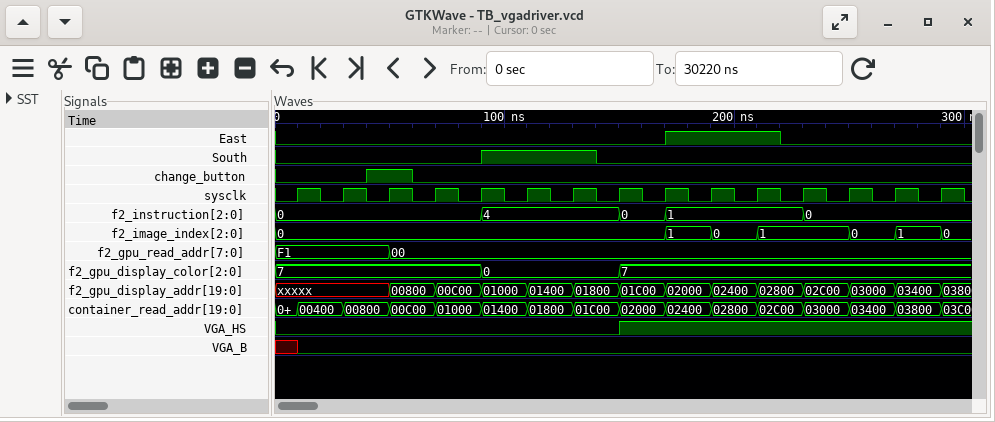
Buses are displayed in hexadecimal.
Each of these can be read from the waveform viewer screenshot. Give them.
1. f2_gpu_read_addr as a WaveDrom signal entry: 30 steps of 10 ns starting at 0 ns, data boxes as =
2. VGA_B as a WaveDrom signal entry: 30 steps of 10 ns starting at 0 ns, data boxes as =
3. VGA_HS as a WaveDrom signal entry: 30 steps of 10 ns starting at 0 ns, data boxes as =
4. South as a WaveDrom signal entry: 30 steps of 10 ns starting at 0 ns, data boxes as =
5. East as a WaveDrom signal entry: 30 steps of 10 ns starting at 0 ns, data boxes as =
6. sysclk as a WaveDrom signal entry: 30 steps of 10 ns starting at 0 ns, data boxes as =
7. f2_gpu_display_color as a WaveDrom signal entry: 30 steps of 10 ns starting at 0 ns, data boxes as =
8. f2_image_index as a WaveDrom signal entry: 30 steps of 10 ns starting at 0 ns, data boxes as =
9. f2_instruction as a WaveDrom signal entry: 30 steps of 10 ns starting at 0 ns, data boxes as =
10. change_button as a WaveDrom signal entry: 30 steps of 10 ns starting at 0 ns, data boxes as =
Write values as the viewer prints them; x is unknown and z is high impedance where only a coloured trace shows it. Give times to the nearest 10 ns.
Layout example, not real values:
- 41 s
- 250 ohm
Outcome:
- {name: 'f2_gpu_read_addr', wave: '=....=........................', data: 'F1 00'}
- {name: 'VGA_B', wave: 'x0............................'}
- {name: 'VGA_HS', wave: '0..............1..............'}
- {name: 'South', wave: '0........1....0...............'}
- {name: 'East', wave: '0................1....0.......'}
- {name: 'sysclk', wave: '010101010101010101010101010101'}
- {name: 'f2_gpu_display_color', wave: '=........=.....=..............', data: '7 0 7'}
- {name: 'f2_image_index', wave: '=................=.=.=...=.=.=', data: '0 1 0 1 0 1 0'}
- {name: 'f2_instruction', wave: '=........=.....=.=.....=......', data: '0 4 0 1 0'}
- {name: 'change_button', wave: '0...1.0.......................'}
